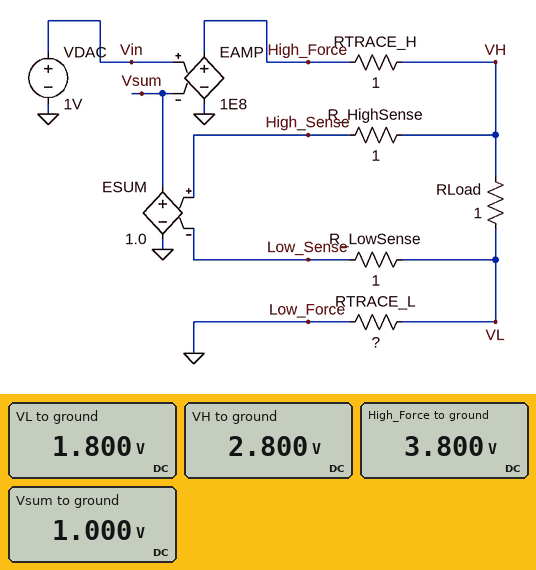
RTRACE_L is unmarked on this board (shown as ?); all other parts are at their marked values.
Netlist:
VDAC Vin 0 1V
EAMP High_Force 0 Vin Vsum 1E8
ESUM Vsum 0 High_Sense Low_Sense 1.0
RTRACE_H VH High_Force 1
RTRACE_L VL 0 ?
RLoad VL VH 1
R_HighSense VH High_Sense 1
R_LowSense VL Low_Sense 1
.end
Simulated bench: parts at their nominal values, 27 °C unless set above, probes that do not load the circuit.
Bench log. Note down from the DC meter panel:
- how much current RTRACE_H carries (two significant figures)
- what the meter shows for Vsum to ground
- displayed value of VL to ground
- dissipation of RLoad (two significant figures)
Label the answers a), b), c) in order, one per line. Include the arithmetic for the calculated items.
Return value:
a) (3.8 V - 2.8 V) / 1 Ω = 1.0 A
b) 1.000 V
c) 1.800 V
d) (2.8 V - 1.8 V)^2 / 1 Ω = 1.0 W
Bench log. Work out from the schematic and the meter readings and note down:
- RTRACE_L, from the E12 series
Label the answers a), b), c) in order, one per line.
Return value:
a) 1.8 Ω
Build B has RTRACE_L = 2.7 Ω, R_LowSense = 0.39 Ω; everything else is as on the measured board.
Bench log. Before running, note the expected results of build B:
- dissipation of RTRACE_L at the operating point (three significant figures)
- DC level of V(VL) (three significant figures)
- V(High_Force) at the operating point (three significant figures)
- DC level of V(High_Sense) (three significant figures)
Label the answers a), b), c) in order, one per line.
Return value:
a) 2.70 W
b) 2.70 V
c) 4.70 V
d) 3.70 V
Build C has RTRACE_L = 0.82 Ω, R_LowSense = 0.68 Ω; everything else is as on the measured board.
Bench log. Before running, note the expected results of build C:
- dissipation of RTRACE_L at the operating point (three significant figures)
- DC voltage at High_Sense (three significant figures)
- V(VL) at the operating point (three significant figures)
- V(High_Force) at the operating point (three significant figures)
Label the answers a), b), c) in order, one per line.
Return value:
a) 820 mW
b) 1.82 V
c) 820 mV
d) 2.82 V
